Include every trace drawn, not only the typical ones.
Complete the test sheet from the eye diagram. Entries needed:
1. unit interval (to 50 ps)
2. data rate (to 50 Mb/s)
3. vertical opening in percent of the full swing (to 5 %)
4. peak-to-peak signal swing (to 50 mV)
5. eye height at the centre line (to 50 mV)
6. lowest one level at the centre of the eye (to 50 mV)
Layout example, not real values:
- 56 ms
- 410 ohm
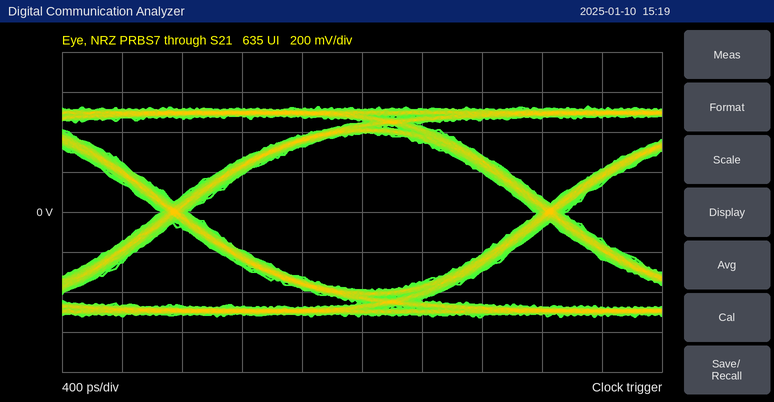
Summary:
- 2.50 ns
- 400 Mb/s
- 75 %
- 1.05 V
- 800 mV
- 400 mV
